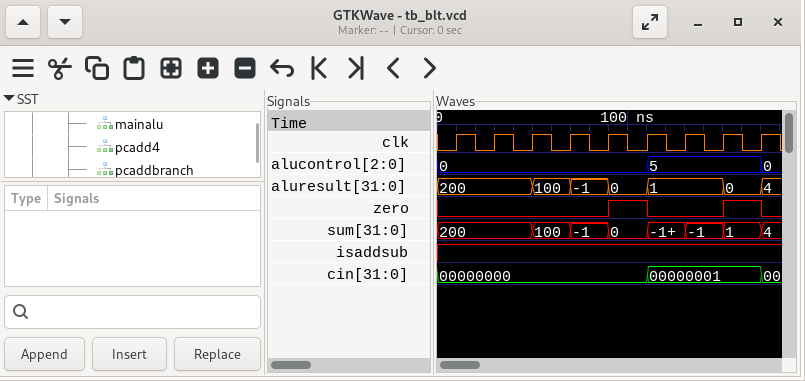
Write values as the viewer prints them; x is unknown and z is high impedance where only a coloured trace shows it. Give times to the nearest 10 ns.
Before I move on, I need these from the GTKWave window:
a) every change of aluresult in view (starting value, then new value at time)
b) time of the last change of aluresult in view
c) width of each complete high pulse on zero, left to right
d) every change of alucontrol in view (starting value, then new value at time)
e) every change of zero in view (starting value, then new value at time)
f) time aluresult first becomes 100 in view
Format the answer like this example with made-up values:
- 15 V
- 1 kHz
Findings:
- 200, 100 at 50 ns, -1 at 70 ns, 0 at 90 ns, 1 at 110 ns, 0 at 150 ns, 4 at 170 ns
- 170 ns
- 20 ns, 20 ns
- 0, 5 at 110 ns, 0 at 170 ns
- 0, 1 at 90 ns, 0 at 110 ns, 1 at 150 ns, 0 at 170 ns
- 50 ns
